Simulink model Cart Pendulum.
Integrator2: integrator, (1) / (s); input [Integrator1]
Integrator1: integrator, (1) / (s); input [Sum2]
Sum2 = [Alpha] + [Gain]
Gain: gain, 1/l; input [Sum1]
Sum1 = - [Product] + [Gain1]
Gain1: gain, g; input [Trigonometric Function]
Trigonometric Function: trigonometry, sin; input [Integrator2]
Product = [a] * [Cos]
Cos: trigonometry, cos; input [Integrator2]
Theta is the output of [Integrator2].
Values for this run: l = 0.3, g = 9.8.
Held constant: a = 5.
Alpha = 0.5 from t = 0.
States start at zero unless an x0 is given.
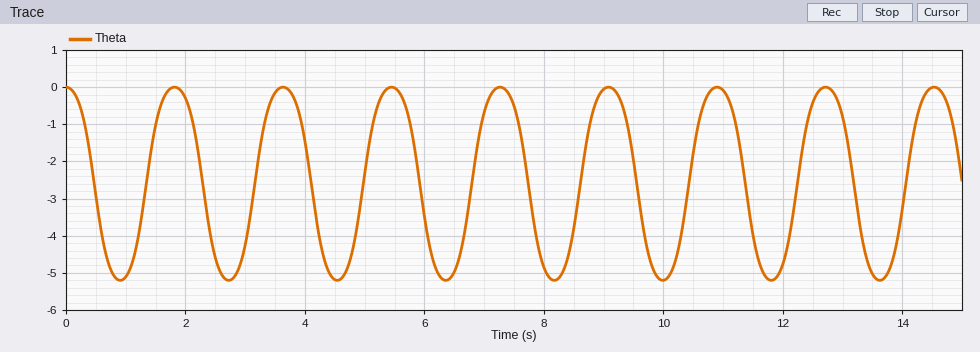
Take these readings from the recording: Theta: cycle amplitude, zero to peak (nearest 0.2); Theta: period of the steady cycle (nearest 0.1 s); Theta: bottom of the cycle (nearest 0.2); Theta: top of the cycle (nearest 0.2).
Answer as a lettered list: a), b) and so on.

a) 2.6
b) 1.8 s
c) -5.2
d) 0.0
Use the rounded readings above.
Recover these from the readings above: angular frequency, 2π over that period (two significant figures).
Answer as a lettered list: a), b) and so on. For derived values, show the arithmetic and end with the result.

a) 2π / 1.8 = 3.5 rad/s
